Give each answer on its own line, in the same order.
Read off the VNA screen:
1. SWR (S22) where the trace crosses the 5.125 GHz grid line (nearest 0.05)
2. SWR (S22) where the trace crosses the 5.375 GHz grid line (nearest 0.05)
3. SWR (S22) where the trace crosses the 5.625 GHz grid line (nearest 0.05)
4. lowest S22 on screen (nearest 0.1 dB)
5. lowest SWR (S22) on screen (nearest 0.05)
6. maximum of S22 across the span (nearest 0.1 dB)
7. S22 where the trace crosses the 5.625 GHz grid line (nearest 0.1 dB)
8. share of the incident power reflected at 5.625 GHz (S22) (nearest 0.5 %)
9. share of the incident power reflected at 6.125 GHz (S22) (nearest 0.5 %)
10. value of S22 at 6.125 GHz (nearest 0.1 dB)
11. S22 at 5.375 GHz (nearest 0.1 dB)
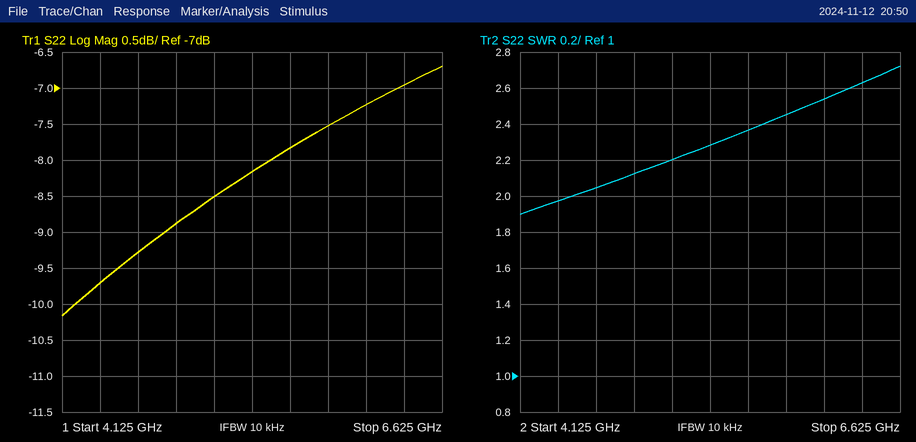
2.20
2.30
2.35
-10.2 dB
1.90
-6.7 dB
-7.8 dB
16.5 %
19.0 %
-7.2 dB
-8.2 dB
